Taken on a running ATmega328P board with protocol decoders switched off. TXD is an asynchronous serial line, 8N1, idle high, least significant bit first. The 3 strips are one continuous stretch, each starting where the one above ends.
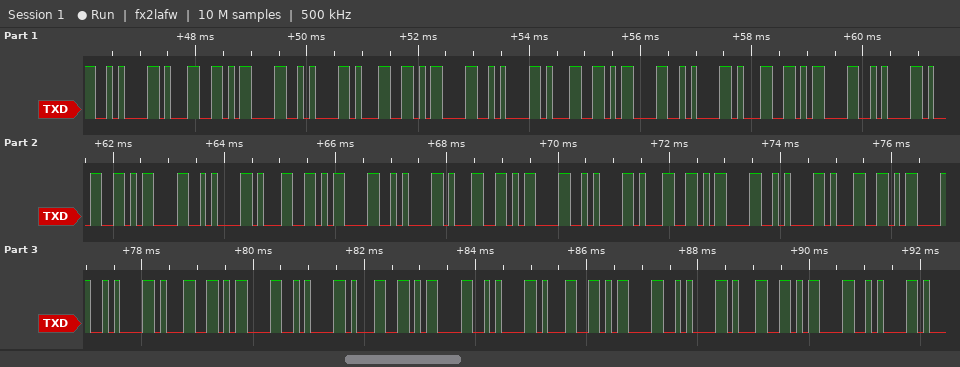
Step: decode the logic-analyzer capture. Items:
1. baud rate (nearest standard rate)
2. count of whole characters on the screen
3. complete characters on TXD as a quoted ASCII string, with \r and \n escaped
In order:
9600 baud
40
"\n1\r\n1\r\n1\r\n1\r\n1\r\n1\r\n1\r\n1\r\n1\r\n1\r\n1\r\n1\r\n1\r\n"
